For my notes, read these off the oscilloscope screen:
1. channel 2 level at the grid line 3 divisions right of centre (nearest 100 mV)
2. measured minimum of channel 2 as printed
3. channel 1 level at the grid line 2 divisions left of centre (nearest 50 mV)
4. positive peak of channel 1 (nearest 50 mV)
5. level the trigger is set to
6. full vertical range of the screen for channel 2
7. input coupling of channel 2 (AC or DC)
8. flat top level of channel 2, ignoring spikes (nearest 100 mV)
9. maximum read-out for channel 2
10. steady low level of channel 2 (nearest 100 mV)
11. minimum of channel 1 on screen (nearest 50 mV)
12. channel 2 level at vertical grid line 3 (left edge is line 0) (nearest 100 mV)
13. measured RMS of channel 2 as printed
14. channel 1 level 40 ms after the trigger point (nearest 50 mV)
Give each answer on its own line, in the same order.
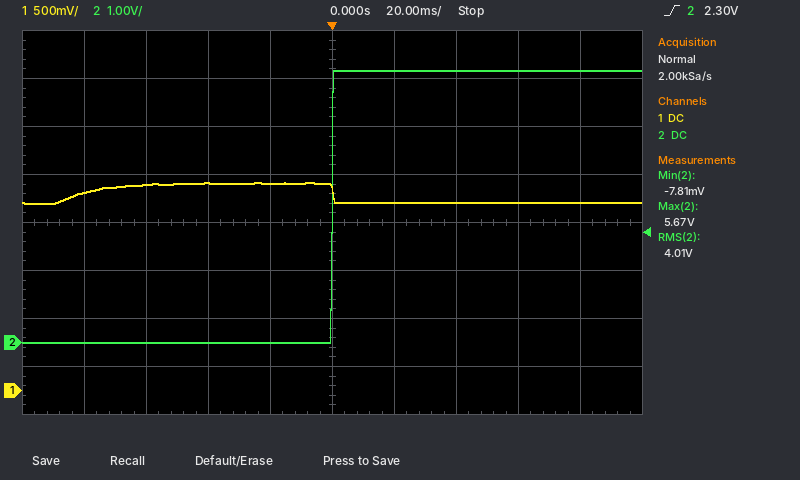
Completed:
5.7 V
-7.81 mV
2.15 V
2.15 V
2.30 V
8 V
DC
5.7 V
5.67 V
0.0 V
1.95 V
0.0 V
4.01 V
1.95 V
